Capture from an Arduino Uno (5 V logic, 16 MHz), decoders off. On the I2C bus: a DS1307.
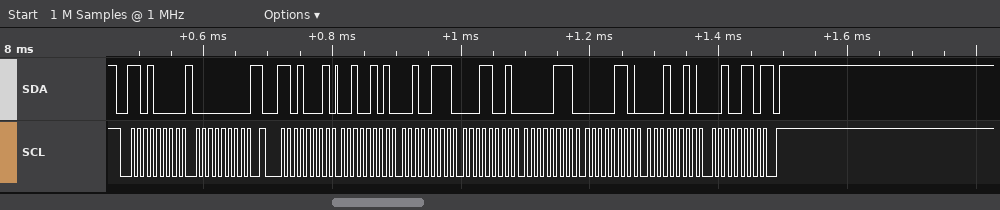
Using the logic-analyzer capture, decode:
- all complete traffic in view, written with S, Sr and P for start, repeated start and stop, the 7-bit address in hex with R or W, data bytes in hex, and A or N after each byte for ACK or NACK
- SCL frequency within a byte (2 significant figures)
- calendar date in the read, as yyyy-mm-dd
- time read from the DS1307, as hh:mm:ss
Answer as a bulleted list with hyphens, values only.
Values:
- S 68W A 00 A Sr 68R A 25 A 27 A 19 A 07 A 06 A 12 A 26 N P
- 100 kHz
- 2026-12-06
- 19:27:25
